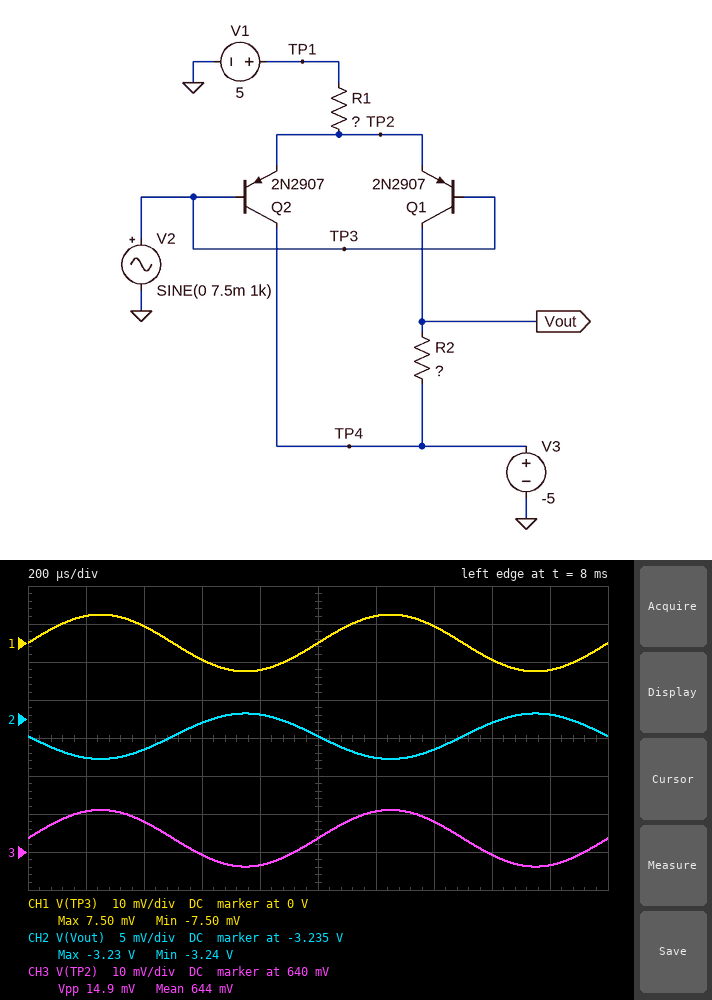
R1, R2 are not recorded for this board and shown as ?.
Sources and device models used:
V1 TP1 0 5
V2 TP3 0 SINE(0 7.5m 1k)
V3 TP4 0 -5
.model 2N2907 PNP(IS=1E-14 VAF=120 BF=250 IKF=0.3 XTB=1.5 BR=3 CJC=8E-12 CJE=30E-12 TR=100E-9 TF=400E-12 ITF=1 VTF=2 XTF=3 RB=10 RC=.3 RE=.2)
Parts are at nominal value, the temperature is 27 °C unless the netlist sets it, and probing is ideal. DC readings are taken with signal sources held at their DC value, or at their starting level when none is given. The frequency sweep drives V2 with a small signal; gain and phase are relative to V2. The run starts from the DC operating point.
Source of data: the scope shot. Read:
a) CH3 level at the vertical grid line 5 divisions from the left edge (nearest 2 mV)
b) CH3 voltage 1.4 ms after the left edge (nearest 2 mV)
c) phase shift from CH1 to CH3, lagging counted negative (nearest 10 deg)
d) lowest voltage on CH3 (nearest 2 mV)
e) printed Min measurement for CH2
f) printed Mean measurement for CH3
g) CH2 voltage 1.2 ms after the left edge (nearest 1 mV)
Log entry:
644 mV
648 mV
0 deg
636 mV
-3.24 V
644 mV
-3.240 V
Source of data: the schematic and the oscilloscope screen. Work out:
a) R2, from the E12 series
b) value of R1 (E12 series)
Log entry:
2.7 kΩ
3.3 kΩ
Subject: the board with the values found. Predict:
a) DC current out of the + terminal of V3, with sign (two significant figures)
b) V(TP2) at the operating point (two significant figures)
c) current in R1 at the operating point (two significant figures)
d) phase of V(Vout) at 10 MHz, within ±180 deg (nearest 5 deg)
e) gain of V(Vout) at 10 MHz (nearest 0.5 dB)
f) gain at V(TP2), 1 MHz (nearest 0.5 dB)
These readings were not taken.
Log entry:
-1.3 mA
640 mV
1.3 mA
75 deg
-3.0 dB
0 dB
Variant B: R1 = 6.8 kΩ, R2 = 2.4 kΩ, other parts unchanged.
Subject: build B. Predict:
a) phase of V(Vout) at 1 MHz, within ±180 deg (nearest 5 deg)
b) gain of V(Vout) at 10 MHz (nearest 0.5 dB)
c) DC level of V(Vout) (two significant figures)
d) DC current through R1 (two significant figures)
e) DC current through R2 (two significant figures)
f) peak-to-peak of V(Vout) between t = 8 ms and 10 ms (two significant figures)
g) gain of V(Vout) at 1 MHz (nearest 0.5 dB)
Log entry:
155 deg
-4.5 dB
-4.2 V
640 µA
320 µA
2.6 mV
-14.5 dB
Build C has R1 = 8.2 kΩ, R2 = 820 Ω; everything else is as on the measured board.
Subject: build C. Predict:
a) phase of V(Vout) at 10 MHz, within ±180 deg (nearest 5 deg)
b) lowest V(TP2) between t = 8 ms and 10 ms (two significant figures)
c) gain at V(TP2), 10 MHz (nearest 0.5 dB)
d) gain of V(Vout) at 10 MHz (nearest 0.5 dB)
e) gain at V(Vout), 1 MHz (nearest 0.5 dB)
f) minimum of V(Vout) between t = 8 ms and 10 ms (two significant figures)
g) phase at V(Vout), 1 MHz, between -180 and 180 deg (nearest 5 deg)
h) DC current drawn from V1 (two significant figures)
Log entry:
90 deg
610 mV
0 dB
-13.0 dB
-25.5 dB
-4.8 V
155 deg
530 µA
